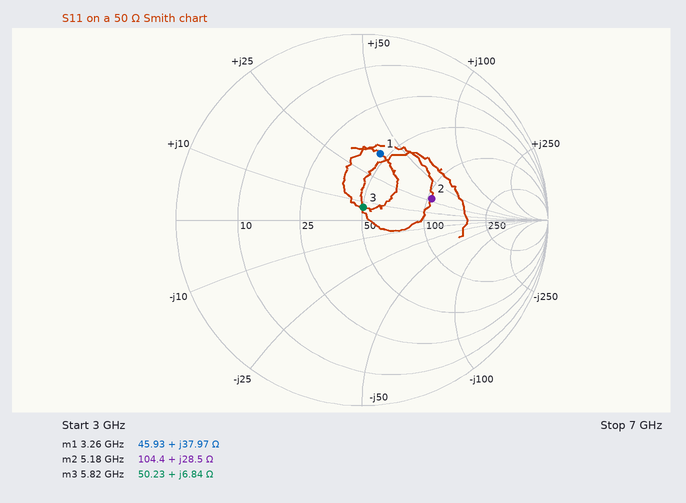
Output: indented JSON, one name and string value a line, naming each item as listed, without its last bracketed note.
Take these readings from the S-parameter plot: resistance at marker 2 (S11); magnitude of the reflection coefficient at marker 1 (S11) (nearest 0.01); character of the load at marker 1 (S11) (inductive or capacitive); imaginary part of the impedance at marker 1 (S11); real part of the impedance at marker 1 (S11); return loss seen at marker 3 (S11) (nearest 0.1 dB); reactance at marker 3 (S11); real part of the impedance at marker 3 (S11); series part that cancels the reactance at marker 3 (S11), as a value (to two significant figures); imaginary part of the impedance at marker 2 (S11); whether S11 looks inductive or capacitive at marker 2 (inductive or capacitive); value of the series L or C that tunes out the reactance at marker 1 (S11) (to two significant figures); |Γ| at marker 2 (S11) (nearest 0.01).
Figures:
{
  "resistance at marker 2": "104.4 Ω",
  "magnitude of the reflection coefficient at marker 1 (S11)": "0.37",
  "character of the load at marker 1 (S11)": "inductive",
  "imaginary part of the impedance at marker 1": "+37.97 Ω",
  "real part of the impedance at marker 1": "45.93 Ω",
  "return loss seen at marker 3 (S11)": "23.3 dB",
  "reactance at marker 3": "+6.84 Ω",
  "real part of the impedance at marker 3": "50.23 Ω",
  "series part that cancels the reactance at marker 3 (S11), as a value": "4.0 pF",
  "imaginary part of the impedance at marker 2": "+28.5 Ω",
  "whether S11 looks inductive or capacitive at marker 2": "inductive",
  "value of the series L or C that tunes out the reactance at marker 1 (S11)": "1.3 pF",
  "|Γ| at marker 2 (S11)": "0.39"
}
